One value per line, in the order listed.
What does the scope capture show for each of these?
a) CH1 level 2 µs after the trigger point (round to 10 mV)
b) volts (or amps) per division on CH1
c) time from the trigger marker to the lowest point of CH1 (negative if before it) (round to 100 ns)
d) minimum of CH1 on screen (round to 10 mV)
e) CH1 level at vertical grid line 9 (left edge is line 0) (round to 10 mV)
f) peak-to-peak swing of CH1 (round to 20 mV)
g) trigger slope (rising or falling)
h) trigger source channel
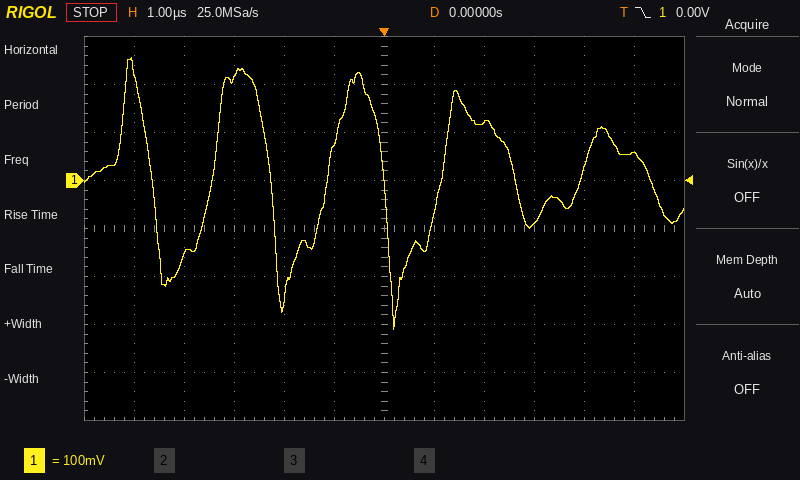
120 mV
100 mV
+200 ns
-310 mV
-90 mV
560 mV
falling
CH1
